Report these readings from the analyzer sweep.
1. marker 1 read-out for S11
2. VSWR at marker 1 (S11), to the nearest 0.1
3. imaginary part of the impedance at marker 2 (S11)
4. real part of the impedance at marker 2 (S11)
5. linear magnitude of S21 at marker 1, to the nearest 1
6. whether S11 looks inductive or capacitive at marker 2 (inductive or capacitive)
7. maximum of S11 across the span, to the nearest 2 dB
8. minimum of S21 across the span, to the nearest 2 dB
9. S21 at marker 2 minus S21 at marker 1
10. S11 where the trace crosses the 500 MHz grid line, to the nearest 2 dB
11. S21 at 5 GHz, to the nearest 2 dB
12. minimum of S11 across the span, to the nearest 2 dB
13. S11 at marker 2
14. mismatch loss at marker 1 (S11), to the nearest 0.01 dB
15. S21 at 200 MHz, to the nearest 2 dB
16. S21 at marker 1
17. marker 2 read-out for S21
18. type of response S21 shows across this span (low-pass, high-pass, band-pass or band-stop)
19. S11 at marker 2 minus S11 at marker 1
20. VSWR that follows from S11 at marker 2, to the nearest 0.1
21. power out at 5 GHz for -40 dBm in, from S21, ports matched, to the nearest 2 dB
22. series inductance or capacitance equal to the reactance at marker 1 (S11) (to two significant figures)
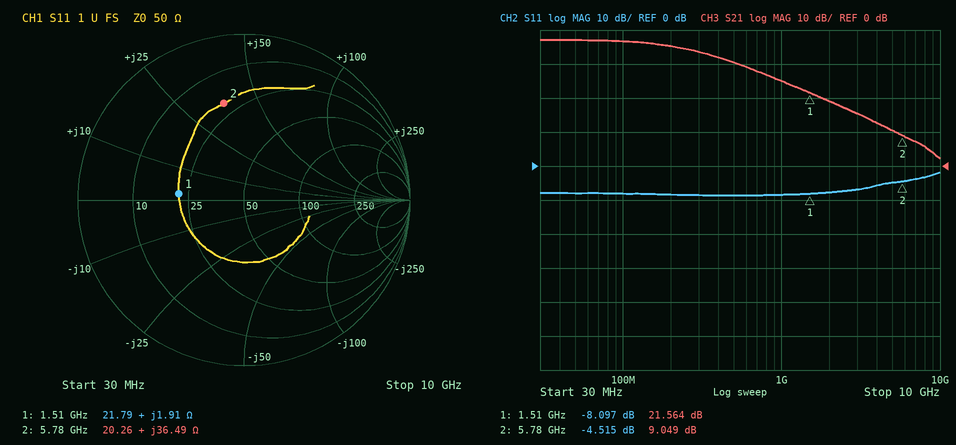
-8.097 dB
2.3
+36.49 Ω
20.26 Ω
12
inductive
-2 dB
2 dB
-12.515 dB
-8 dB
10 dB
-8 dB
-4.515 dB
0.73 dB
36 dB
21.564 dB
9.049 dB
low-pass
3.582 dB
3.9
-30 dBm
200 pH
